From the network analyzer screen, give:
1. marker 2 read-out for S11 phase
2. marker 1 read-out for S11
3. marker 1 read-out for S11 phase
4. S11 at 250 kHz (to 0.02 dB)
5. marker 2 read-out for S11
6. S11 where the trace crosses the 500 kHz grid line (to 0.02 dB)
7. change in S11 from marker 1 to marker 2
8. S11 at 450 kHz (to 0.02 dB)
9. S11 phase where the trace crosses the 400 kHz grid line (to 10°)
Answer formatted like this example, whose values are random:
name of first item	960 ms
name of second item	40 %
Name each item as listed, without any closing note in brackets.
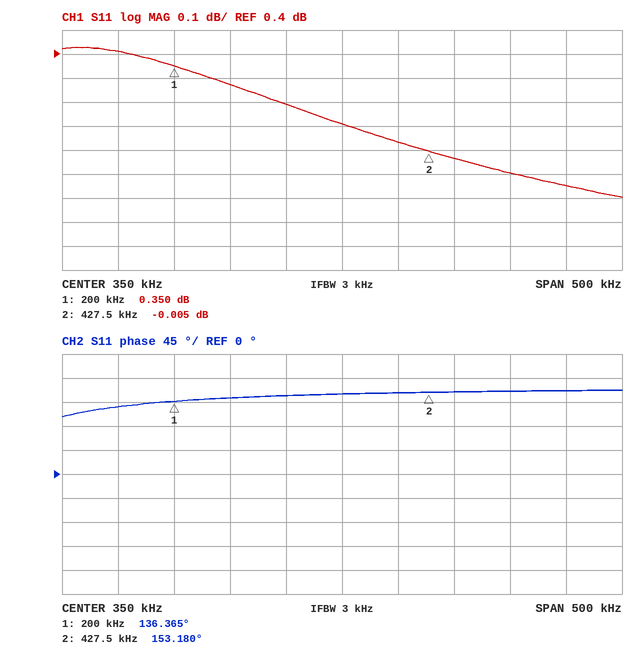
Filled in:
marker 2 read-out for S11 phase	153.180°
marker 1 read-out for S11	0.350 dB
marker 1 read-out for S11 phase	136.365°
S11 at 250 kHz	0.28 dB
marker 2 read-out for S11	-0.005 dB
S11 where the trace crosses the 500 kHz grid line	-0.10 dB
change in S11 from marker 1 to marker 2	-0.355 dB
S11 at 450 kHz	-0.04 dB
S11 phase where the trace crosses the 400 kHz grid line	150°
